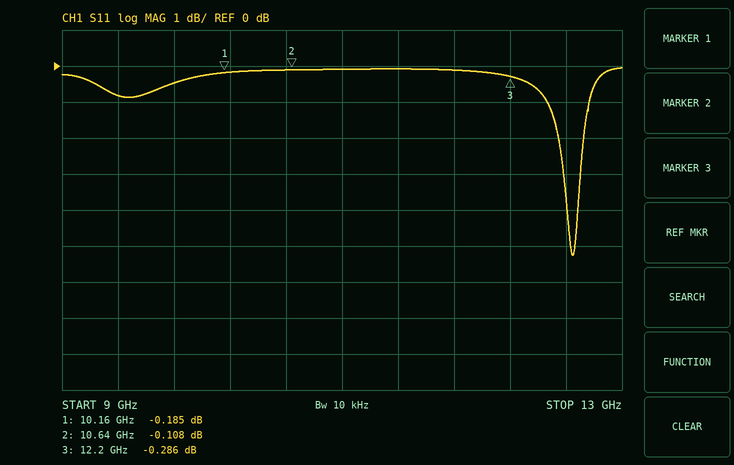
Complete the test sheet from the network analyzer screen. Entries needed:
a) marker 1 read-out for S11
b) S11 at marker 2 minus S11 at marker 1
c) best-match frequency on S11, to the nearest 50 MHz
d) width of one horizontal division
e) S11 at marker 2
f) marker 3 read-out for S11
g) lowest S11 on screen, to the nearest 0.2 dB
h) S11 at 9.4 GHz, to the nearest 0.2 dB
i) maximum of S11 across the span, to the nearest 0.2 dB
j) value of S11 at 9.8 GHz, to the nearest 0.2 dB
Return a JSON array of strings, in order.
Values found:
["-0.185 dB", "0.077 dB", "12.65 GHz", "400 MHz", "-0.108 dB", "-0.286 dB", "-5.2 dB", "-0.8 dB", "0.0 dB", "-0.4 dB"]
